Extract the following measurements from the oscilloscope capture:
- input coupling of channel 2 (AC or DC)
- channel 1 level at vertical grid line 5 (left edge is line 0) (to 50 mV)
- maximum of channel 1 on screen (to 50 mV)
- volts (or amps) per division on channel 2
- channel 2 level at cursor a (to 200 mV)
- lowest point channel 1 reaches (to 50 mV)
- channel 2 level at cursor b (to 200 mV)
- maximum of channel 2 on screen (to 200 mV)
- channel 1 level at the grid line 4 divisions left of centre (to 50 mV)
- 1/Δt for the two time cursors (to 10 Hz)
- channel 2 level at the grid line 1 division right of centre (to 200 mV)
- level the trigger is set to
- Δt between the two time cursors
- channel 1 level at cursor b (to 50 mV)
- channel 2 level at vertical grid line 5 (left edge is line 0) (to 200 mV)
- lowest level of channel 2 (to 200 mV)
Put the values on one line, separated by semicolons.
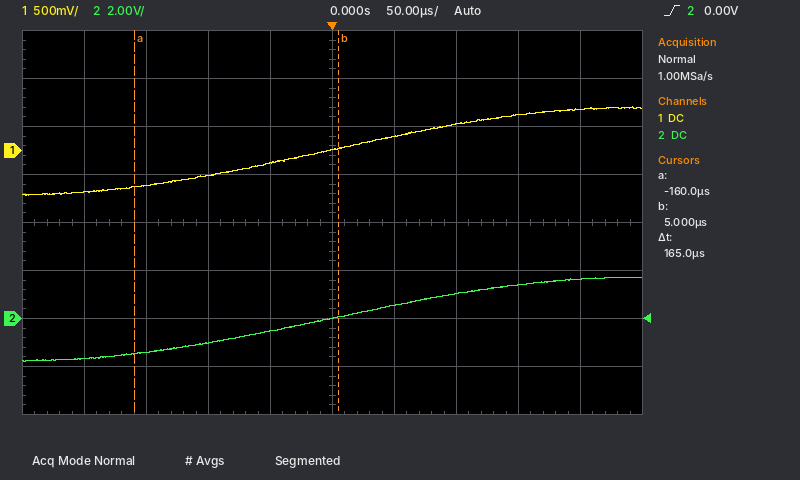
DC; 0 mV; 450 mV; 2 V; -1.4 V; -450 mV; 0.0 V; 1.8 V; -450 mV; 6.06 kHz; 600 mV; 0.00 V; 165 µs; 0 mV; 0.0 V; -1.8 V
